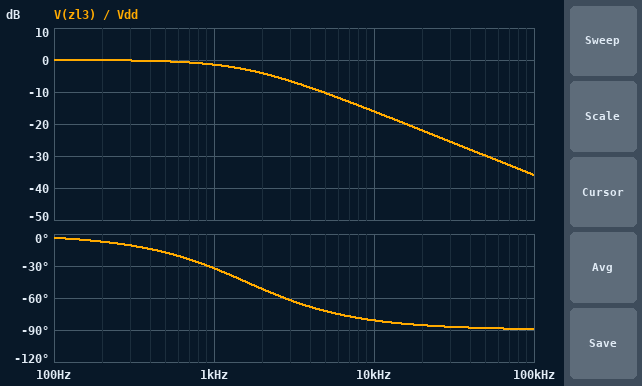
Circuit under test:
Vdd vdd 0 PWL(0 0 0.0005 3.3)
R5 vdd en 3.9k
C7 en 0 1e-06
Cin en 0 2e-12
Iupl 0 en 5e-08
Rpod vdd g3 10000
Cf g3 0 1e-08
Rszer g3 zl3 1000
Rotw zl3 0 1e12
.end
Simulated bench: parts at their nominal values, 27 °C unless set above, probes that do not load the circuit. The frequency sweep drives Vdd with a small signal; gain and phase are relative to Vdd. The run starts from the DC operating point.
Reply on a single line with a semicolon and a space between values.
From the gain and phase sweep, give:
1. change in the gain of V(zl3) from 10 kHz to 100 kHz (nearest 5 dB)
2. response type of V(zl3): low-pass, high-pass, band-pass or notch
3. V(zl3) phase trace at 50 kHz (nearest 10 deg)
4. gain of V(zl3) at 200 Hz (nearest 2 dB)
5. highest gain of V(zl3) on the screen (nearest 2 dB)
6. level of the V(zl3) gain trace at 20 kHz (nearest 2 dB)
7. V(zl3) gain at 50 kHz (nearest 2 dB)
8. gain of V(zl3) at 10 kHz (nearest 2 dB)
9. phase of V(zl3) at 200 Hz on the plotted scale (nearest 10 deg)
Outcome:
-20 dB; low-pass; -90 deg; 0 dB; 0 dB; -22 dB; -30 dB; -16 dB; -10 deg
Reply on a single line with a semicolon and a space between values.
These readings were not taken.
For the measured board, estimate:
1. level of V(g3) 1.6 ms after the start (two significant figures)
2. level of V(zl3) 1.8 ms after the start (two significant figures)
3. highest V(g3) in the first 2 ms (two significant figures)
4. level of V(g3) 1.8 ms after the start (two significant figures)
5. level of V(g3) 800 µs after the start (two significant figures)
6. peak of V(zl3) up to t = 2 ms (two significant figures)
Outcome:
3.3 V; 3.3 V; 3.3 V; 3.3 V; 3.3 V; 3.3 V
